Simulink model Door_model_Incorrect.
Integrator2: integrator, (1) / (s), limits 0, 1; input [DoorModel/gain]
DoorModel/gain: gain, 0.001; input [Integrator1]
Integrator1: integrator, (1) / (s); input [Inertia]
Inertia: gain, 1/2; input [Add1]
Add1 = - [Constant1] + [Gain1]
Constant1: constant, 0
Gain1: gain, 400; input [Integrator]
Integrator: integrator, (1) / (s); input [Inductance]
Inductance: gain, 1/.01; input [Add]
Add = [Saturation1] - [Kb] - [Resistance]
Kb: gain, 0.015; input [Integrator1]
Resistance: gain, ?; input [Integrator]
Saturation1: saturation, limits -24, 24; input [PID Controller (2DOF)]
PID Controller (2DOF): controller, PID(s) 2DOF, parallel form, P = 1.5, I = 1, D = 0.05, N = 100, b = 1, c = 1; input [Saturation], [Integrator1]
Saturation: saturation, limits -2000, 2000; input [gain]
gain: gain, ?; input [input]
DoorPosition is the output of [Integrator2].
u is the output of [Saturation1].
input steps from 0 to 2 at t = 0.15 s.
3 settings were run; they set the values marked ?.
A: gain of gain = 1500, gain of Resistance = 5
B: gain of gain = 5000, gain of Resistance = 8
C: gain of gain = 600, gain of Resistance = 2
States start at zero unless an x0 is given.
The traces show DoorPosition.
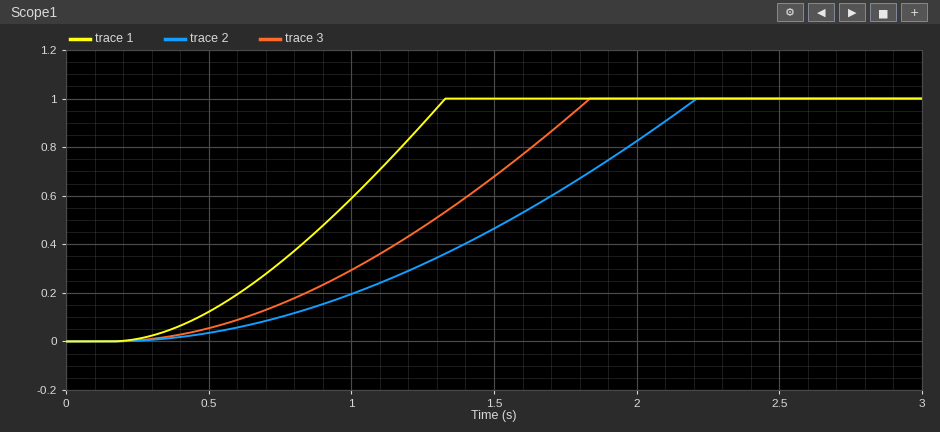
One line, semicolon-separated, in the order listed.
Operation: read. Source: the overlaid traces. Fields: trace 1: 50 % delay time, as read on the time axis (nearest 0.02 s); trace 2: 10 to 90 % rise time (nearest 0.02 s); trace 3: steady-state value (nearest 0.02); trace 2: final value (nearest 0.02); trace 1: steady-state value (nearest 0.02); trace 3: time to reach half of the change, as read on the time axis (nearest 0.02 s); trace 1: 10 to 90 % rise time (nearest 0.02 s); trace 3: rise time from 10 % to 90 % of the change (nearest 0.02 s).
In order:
0.92 s; 1.34 s; 1.00; 1.00; 1.00; 1.28 s; 0.78 s; 1.10 s
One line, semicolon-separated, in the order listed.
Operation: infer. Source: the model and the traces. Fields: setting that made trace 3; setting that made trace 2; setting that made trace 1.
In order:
A; B; C
